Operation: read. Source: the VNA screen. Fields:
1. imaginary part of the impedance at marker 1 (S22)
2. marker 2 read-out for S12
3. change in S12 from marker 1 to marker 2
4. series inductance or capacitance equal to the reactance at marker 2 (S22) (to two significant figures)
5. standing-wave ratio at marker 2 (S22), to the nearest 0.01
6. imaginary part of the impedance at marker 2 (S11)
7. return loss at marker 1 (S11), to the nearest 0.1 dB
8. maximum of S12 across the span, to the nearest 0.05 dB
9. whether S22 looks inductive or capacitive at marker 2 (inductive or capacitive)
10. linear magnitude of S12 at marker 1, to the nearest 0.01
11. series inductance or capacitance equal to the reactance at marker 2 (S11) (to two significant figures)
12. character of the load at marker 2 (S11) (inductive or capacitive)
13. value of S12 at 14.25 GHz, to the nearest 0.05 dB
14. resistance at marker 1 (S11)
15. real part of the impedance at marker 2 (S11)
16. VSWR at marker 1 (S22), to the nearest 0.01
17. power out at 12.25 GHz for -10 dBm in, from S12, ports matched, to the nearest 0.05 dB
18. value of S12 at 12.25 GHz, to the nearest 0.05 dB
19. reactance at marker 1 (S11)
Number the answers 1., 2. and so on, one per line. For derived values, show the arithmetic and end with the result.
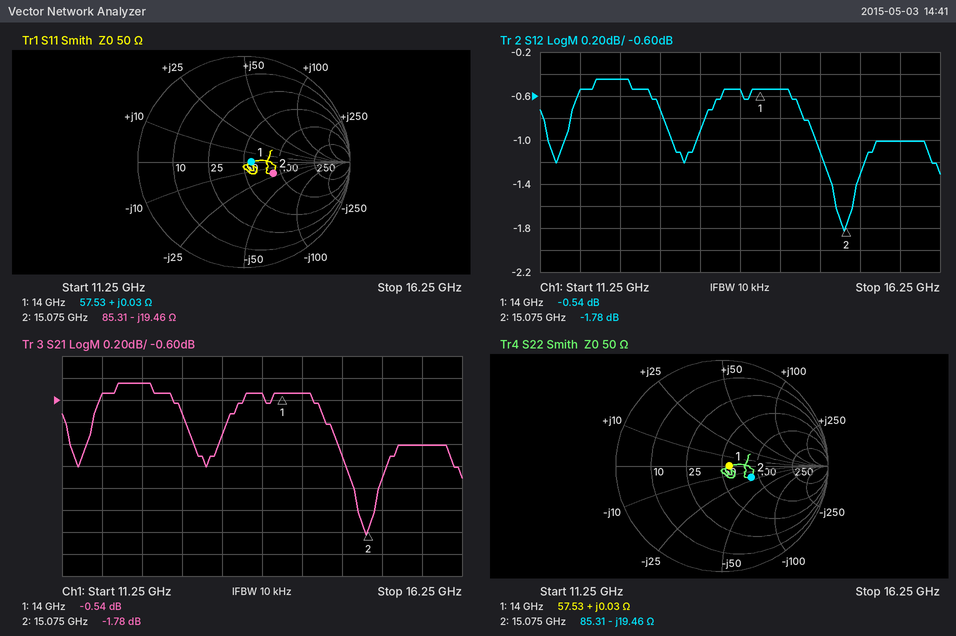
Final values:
1. +0.03 Ω
2. -1.78 dB
3. -1.78 − (-0.54) = -1.24 dB
4. C = 1/(2π × 15.075 GHz × 19.46 Ω) ≈ 543 fF, so 540 fF to two significant figures
5. 1.84
6. -19.46 Ω
7. 23.1 dB
8. -0.45 dB
9. capacitive
10. 10^(-0.54/20) ≈ 0.94
11. C = 1/(2π × 15.075 GHz × 19.46 Ω) ≈ 543 fF, so 540 fF to two significant figures
12. capacitive
13. -0.55 dB
14. 57.53 Ω
15. 85.31 Ω
16. 1.15
17. -10 dBm + (-0.45 dB) = -10.45 dBm
18. -0.45 dB
19. +0.03 Ω
